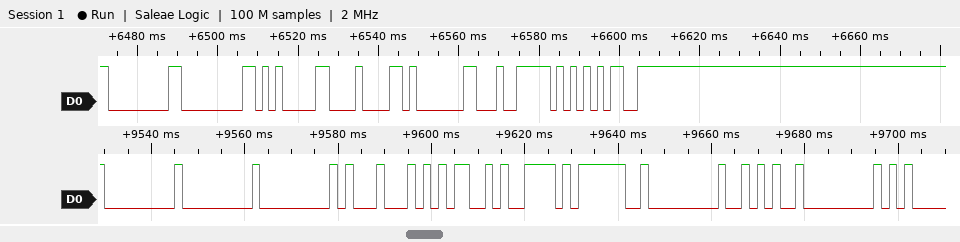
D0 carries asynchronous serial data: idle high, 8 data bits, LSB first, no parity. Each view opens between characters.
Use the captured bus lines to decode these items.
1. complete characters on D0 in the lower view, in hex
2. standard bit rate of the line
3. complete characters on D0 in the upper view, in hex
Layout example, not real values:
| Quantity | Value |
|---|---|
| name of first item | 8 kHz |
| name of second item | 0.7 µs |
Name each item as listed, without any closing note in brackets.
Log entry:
| Quantity | Value |
|---|---|
| complete characters on D0 in the lower view, in hex | 00, 00, 00, 11, 35, 79, 3F, 00, 2A, 00 |
| standard bit rate of the line | 600 baud |
| complete characters on D0 in the upper view, in hex | 00, 00, 05, 08, 01, E4, 55, FE |
